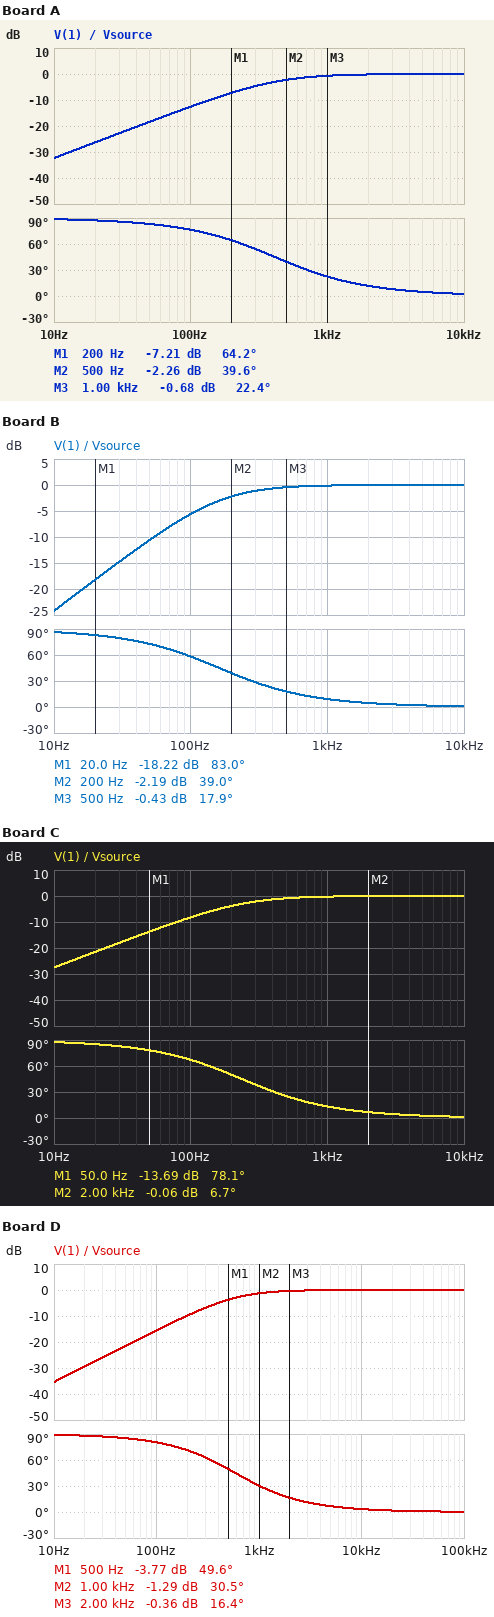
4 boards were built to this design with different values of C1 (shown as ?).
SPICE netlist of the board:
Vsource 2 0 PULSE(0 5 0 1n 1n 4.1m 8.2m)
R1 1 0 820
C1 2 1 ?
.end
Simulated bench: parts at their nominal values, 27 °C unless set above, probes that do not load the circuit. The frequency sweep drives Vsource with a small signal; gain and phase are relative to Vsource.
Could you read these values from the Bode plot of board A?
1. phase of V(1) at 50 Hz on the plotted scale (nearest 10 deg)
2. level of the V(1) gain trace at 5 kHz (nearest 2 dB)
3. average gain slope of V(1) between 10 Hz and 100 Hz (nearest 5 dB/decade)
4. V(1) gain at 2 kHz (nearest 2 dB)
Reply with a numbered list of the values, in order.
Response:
1. 80 deg
2. 0 dB
3. 20 dB/decade
4. 0 dB
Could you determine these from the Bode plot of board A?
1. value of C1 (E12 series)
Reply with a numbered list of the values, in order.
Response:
1. 470 nF
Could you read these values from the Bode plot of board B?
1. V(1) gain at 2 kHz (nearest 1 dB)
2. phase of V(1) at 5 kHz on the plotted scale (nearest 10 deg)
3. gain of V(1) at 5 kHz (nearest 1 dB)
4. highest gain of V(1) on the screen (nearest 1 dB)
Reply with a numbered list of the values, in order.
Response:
1. 0 dB
2. 0 deg
3. 0 dB
4. 0 dB
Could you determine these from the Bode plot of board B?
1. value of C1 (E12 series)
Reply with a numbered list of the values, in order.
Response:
1. 1.2 µF
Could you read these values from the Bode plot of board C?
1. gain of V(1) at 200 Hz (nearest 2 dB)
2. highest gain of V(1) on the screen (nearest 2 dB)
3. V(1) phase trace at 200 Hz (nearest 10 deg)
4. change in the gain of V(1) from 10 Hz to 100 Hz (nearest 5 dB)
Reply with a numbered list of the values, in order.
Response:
1. -4 dB
2. 0 dB
3. 50 deg
4. 20 dB
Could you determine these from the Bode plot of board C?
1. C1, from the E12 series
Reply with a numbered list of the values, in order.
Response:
1. 820 nF
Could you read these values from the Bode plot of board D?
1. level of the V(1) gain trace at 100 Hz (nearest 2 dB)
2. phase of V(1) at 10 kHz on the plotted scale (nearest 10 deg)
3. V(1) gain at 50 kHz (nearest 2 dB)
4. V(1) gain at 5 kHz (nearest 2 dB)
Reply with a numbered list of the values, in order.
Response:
1. -16 dB
2. 0 deg
3. 0 dB
4. 0 dB
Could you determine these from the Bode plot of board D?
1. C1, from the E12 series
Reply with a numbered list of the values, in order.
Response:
1. 330 nF
